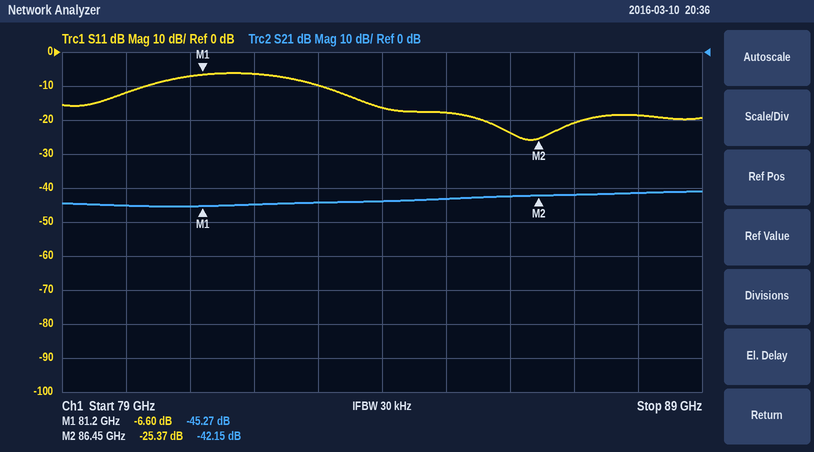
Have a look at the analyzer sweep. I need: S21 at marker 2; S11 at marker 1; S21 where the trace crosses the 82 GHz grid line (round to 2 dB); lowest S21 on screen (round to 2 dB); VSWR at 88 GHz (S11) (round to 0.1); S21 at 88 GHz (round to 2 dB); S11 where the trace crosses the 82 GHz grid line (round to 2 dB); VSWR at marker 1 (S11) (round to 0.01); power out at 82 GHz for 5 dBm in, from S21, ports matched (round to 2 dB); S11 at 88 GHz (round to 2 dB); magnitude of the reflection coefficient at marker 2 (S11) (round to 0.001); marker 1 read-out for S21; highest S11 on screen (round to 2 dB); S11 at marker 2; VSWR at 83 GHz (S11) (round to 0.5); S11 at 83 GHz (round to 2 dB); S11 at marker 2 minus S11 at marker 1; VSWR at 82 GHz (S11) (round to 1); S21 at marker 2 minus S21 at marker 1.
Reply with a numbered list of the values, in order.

1. -42.15 dB
2. -6.60 dB
3. -44 dB
4. -46 dB
5. 1.3
6. -42 dB
7. -6 dB
8. 2.76
9. -40 dBm
10. -18 dB
11. 0.054
12. -45.27 dB
13. -6 dB
14. -25.37 dB
15. 2.0
16. -10 dB
17. -18.77 dB
18. 3
19. 3.12 dB
